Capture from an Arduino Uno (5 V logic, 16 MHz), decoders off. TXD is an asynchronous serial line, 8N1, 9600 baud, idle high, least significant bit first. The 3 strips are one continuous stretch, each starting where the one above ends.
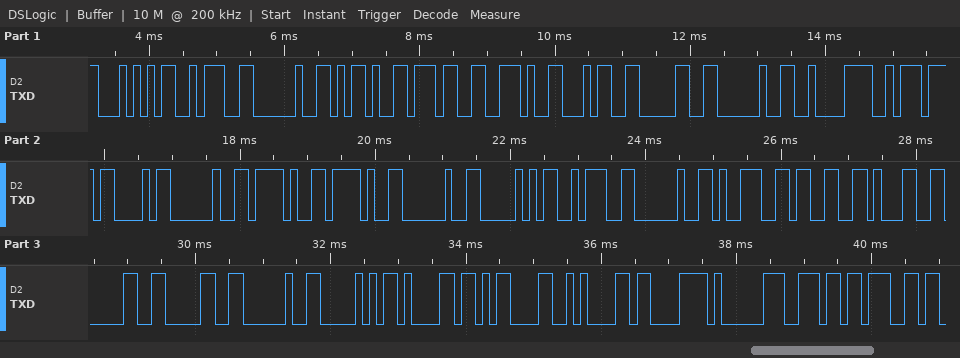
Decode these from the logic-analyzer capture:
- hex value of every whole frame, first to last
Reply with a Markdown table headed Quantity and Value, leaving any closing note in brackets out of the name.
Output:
| Quantity | Value |
|---|---|
| hex value of every whole frame, first to last | 54 3A 20 2D 37 2E 34 30 20 C2 BA 43 20 2F 2F 20 50 3A 20 39 33 31 30 30 20 50 61 0D 0A C3 81 6E 67 |
